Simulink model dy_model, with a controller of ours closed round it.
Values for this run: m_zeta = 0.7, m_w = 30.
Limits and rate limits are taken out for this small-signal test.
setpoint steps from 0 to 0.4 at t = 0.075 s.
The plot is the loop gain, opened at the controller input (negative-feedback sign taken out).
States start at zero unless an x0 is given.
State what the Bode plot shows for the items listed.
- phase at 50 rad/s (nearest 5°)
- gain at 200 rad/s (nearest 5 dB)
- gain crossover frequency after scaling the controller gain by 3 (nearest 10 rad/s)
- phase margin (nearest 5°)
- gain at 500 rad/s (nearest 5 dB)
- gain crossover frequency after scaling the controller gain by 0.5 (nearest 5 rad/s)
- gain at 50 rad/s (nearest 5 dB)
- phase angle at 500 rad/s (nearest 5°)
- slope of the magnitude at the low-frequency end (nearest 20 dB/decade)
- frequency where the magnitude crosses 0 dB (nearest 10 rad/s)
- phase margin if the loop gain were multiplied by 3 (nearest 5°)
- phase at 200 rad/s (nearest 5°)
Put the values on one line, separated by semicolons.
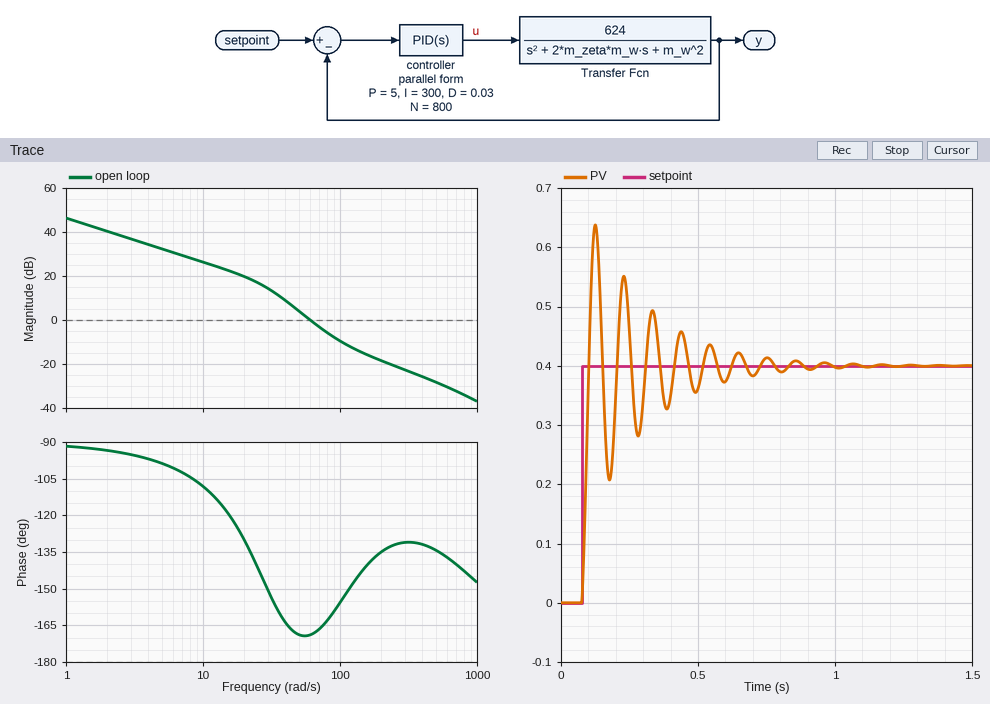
-170°; -20 dB; 100 rad/s; 10°; -30 dB; 45 rad/s; 5 dB; -135°; -20 dB/decade; 60 rad/s; 25°; -135°
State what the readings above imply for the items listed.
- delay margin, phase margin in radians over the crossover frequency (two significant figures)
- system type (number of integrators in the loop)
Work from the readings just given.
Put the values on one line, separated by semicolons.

0.0029 s; 1
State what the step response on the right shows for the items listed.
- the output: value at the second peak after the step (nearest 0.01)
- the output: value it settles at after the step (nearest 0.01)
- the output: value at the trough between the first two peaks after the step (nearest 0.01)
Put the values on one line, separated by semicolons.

0.55; 0.40; 0.21
